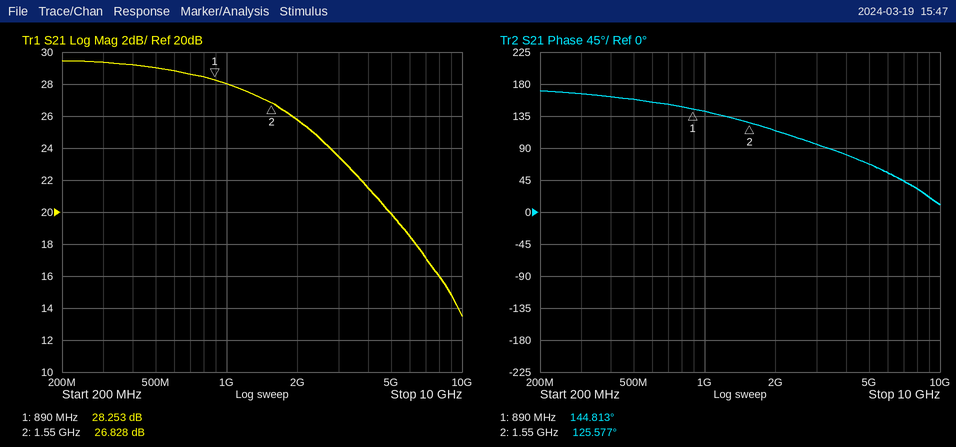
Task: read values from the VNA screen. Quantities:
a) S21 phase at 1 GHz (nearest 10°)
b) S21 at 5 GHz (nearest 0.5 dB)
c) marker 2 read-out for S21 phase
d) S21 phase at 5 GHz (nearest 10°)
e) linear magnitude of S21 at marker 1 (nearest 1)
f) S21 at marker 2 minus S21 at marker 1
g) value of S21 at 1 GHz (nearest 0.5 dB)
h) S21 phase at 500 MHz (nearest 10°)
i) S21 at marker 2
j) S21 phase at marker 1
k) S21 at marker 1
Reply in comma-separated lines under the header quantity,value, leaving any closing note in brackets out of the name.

quantity,value
S21 phase at 1 GHz,140°
S21 at 5 GHz,20.0 dB
marker 2 read-out for S21 phase,125.577°
S21 phase at 5 GHz,70°
linear magnitude of S21 at marker 1,26
S21 at marker 2 minus S21 at marker 1,-1.425 dB
value of S21 at 1 GHz,28.0 dB
S21 phase at 500 MHz,160°
S21 at marker 2,26.828 dB
S21 phase at marker 1,144.813°
S21 at marker 1,28.253 dB
